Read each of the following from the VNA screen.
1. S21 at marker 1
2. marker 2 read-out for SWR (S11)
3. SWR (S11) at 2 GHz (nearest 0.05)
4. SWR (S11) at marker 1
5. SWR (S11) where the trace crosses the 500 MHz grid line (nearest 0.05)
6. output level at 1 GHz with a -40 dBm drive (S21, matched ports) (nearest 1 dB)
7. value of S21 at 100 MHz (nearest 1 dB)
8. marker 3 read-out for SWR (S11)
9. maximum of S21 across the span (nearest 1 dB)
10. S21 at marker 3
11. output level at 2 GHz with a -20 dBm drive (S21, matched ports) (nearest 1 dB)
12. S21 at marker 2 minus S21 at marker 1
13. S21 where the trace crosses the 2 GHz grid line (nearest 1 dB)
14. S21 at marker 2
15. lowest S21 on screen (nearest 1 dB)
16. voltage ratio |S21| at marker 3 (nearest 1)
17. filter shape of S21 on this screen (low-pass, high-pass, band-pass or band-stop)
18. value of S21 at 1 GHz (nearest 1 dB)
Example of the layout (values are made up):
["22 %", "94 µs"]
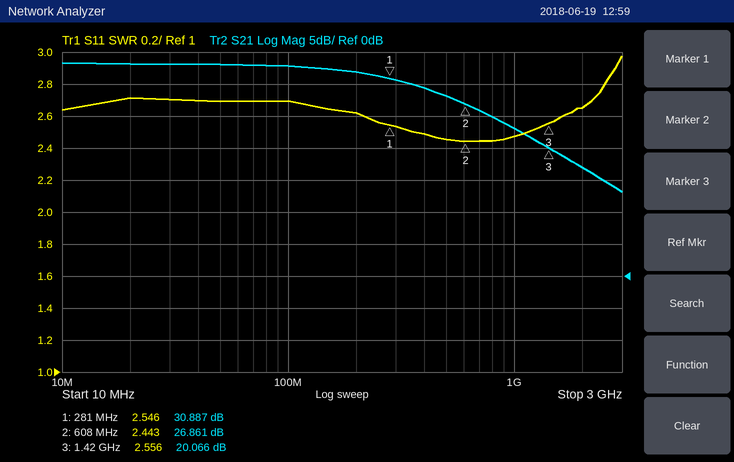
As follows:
["30.887 dB", "2.443", "2.65", "2.546", "2.45", "-17 dBm", "33 dB", "2.556", "33 dB", "20.066 dB", "-3 dBm", "-4.026 dB", "17 dB", "26.861 dB", "13 dB", "10", "low-pass", "23 dB"]
